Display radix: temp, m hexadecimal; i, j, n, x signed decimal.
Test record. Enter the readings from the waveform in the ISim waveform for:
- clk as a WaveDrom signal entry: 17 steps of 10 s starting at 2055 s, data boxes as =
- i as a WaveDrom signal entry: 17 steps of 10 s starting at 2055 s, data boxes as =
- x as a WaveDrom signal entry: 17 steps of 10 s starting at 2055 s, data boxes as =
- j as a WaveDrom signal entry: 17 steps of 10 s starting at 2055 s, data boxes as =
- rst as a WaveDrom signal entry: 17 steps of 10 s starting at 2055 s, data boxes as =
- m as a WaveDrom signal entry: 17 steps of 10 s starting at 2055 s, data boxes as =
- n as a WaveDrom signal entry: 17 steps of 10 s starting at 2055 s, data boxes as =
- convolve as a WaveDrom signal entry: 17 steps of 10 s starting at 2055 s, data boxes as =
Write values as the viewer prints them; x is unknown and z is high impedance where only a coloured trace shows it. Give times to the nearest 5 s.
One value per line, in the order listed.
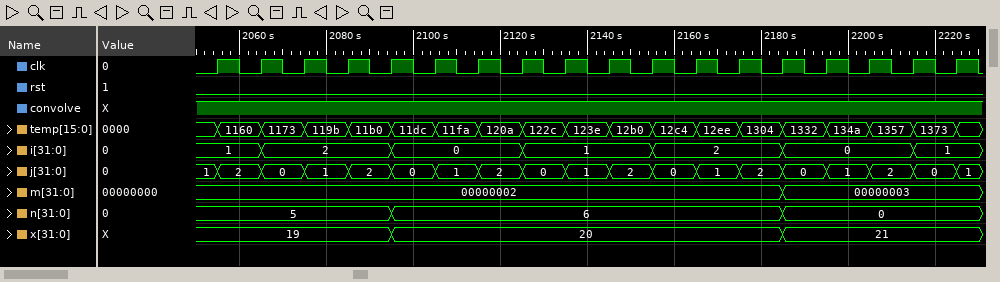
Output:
{name: 'clk', wave: 'p................'}
{name: 'i', wave: '==..=..=..=..=..=', data: '1 2 0 1 2 0 1'}
{name: 'x', wave: '=...=........=...', data: '19 20 21'}
{name: 'j', wave: '=================', data: '2 0 1 2 0 1 2 0 1 2 0 1 2 0 1 2 0'}
{name: 'rst', wave: '0................'}
{name: 'm', wave: '=............=...', data: '00000002 00000003'}
{name: 'n', wave: '=...=........=...', data: '5 6 0'}
{name: 'convolve', wave: '1................'}
